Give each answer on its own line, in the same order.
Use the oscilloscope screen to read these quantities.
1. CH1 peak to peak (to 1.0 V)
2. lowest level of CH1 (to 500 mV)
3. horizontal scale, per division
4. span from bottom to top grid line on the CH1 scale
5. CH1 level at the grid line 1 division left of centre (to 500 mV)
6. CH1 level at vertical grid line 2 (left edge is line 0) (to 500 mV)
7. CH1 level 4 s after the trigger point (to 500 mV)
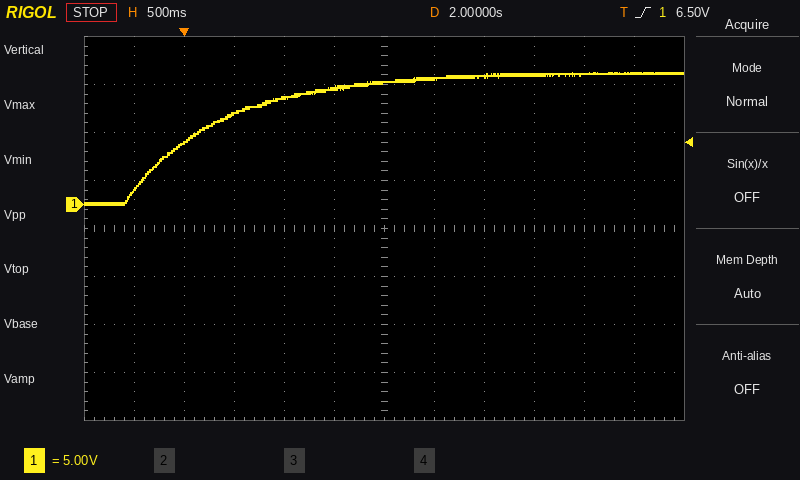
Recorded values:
14.0 V
0.0 V
500 ms
40 V
12.0 V
6.5 V
13.5 V
